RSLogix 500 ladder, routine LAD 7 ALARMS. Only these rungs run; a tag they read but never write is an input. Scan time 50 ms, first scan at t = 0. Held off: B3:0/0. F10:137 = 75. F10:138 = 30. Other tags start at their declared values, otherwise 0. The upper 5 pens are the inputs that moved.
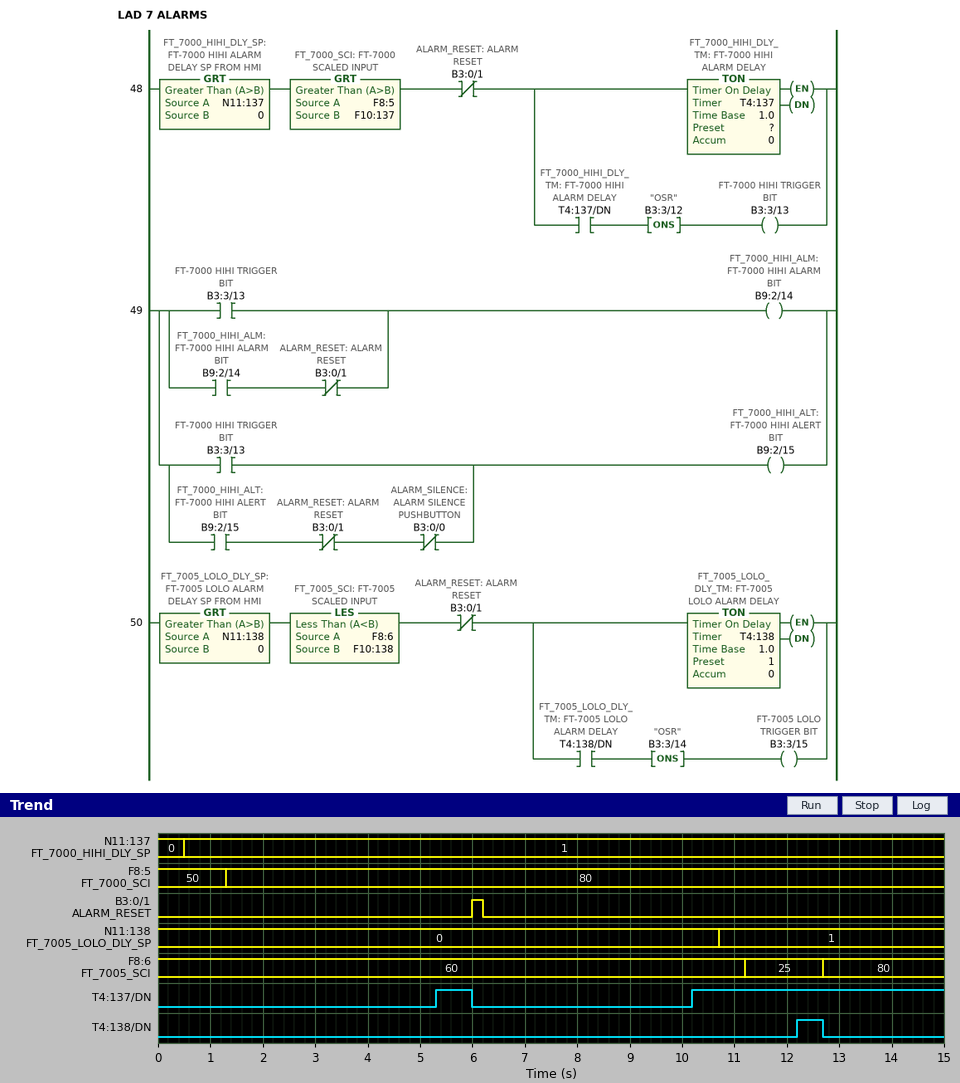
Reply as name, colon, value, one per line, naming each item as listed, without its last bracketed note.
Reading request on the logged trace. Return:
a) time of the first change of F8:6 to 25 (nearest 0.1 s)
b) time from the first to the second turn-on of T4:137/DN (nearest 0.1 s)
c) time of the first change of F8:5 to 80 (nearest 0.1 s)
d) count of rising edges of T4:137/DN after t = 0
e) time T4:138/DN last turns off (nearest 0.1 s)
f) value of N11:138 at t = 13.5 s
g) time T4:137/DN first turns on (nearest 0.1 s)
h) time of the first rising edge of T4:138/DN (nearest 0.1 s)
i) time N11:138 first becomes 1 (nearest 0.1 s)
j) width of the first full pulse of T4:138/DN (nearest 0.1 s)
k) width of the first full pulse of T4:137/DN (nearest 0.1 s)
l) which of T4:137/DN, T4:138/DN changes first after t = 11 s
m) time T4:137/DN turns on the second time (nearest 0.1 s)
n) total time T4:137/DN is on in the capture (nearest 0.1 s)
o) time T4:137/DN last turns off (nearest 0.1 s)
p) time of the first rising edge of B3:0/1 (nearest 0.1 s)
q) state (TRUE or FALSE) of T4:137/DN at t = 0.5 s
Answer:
time of the first change of F8:6 to 25: 11.2 s
time from the first to the second turn-on of T4:137/DN: 4.9 s
time of the first change of F8:5 to 80: 1.3 s
count of rising edges of T4:137/DN after t = 0: 2
time T4:138/DN last turns off: 12.7 s
value of N11:138 at t = 13.5 s: 1
time T4:137/DN first turns on: 5.3 s
time of the first rising edge of T4:138/DN: 12.2 s
time N11:138 first becomes 1: 10.7 s
width of the first full pulse of T4:138/DN: 0.5 s
width of the first full pulse of T4:137/DN: 0.7 s
which of T4:137/DN, T4:138/DN changes first after t = 11 s: T4:138/DN
time T4:137/DN turns on the second time: 10.2 s
total time T4:137/DN is on in the capture: 5.5 s
time T4:137/DN last turns off: 6.0 s
time of the first rising edge of B3:0/1: 6.0 s
state (TRUE or FALSE) of T4:137/DN at t = 0.5 s: FALSE
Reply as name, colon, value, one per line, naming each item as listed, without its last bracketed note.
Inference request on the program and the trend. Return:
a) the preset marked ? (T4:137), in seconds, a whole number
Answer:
the preset marked ? (T4:137), in seconds, a whole number: 4 s
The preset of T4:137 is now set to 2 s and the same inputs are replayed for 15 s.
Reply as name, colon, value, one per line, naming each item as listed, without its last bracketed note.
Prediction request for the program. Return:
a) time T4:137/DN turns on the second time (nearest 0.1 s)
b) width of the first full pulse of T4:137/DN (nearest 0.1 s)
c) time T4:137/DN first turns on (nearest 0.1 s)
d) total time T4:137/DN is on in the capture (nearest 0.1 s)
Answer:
time T4:137/DN turns on the second time: 8.2 s
width of the first full pulse of T4:137/DN: 2.7 s
time T4:137/DN first turns on: 3.3 s
total time T4:137/DN is on in the capture: 9.5 s
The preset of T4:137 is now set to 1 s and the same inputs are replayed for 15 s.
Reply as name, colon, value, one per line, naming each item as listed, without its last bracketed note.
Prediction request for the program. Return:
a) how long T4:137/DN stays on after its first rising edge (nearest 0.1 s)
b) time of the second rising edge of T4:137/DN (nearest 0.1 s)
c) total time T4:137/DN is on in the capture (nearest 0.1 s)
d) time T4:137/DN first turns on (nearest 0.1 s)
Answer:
how long T4:137/DN stays on after its first rising edge: 3.7 s
time of the second rising edge of T4:137/DN: 7.2 s
total time T4:137/DN is on in the capture: 11.5 s
time T4:137/DN first turns on: 2.3 s
